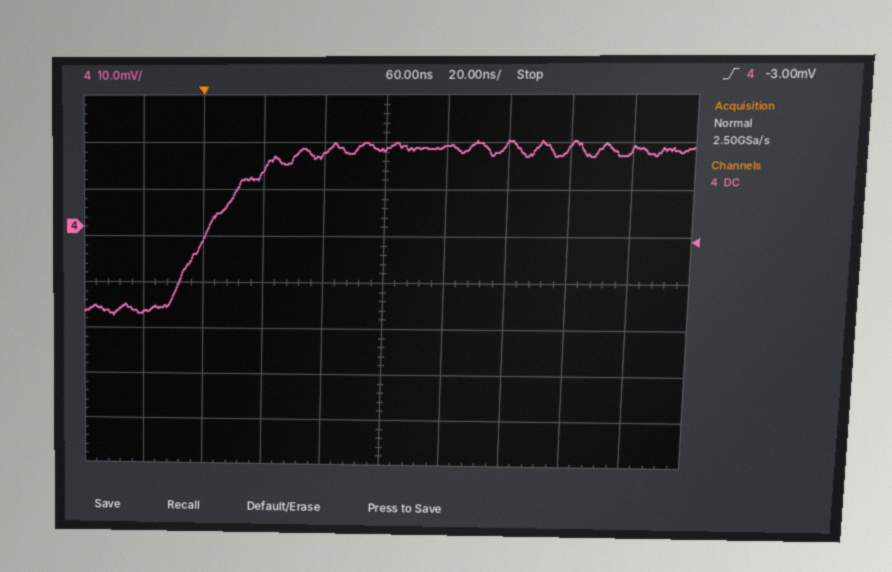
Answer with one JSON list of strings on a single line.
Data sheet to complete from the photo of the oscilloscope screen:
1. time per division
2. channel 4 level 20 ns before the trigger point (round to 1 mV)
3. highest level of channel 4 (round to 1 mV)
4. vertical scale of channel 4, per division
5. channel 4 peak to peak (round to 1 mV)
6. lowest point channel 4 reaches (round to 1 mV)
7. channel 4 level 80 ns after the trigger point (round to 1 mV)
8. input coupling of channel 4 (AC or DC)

["20 ns", "-18 mV", "18 mV", "10 mV", "37 mV", "-19 mV", "17 mV", "DC"]
